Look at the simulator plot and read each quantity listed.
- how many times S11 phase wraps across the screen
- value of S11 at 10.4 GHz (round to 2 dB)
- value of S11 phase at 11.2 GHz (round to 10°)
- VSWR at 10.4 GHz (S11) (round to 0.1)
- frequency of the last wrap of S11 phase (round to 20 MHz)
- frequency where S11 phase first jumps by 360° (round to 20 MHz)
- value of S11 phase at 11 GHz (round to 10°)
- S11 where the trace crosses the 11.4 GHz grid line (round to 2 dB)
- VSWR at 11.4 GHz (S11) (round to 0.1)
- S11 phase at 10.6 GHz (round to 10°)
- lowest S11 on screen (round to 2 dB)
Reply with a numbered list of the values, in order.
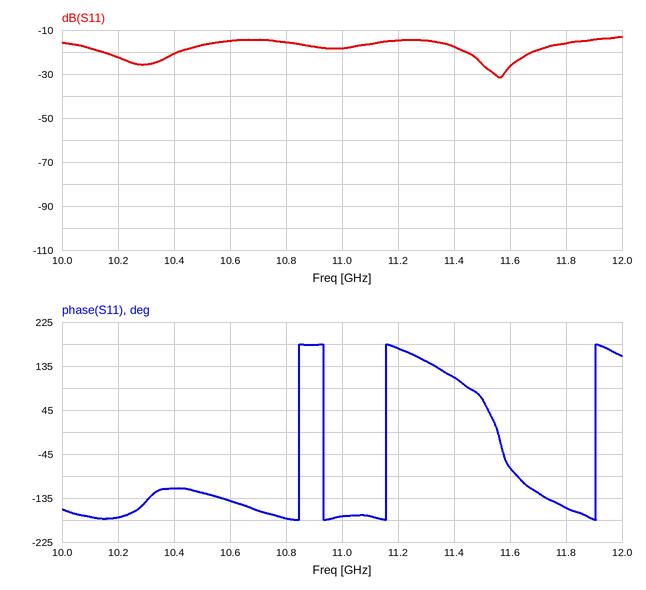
1. 4
2. -20 dB
3. 170°
4. 1.2
5. 11.90 GHz
6. 10.84 GHz
7. -170°
8. -18 dB
9. 1.3
10. -140°
11. -32 dB
